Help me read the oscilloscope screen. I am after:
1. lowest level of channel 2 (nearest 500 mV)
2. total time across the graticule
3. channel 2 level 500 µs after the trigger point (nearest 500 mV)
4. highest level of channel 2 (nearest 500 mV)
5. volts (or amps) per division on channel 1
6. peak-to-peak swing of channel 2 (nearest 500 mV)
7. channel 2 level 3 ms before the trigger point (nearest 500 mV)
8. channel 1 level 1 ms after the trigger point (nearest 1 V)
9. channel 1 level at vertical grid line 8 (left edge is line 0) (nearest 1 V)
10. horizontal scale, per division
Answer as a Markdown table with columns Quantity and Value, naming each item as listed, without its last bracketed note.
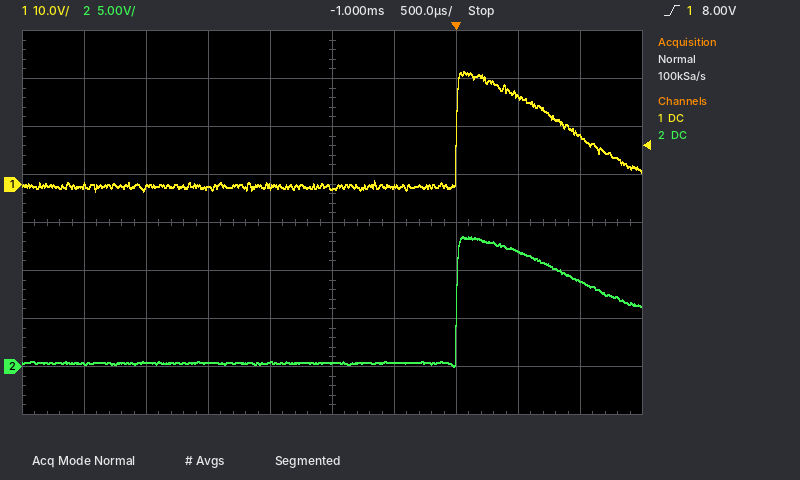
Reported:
| Quantity | Value |
|---|---|
| lowest level of channel 2 | 0.0 V |
| total time across the graticule | 5 ms |
| channel 2 level 500 µs after the trigger point | 12.0 V |
| highest level of channel 2 | 13.5 V |
| volts (or amps) per division on channel 1 | 10 V |
| peak-to-peak swing of channel 2 | 13.5 V |
| channel 2 level 3 ms before the trigger point | 500 mV |
| channel 1 level 1 ms after the trigger point | 10 V |
| channel 1 level at vertical grid line 8 (left edge is line 0) | 18 V |
| horizontal scale, per division | 500 µs |
